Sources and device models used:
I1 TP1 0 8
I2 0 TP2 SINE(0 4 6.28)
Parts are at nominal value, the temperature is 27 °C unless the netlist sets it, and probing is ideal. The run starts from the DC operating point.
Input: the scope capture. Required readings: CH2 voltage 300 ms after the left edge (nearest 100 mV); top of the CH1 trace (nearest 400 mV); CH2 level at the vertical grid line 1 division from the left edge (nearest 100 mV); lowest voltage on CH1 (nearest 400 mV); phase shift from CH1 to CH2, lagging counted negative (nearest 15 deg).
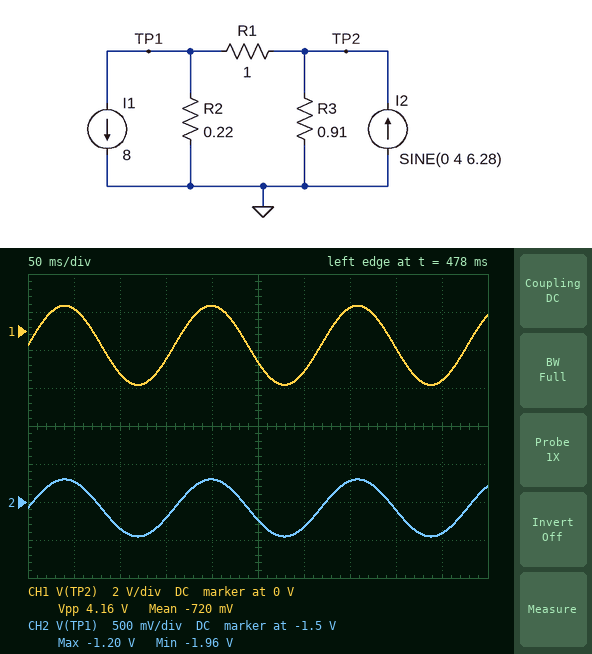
-1.8 V
1.2 V
-1.2 V
-2.8 V
0 deg
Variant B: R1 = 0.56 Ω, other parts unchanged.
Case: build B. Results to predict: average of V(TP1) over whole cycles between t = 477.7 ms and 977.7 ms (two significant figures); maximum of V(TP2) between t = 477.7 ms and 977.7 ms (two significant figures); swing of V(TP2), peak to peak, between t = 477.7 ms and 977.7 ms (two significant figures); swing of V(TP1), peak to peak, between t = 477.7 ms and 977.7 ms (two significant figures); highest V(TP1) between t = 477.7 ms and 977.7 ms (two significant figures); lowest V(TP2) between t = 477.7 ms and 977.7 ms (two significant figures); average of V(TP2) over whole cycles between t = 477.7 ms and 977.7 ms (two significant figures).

-1.5 V
730 mV
3.4 V
950 mV
-1.1 V
-2.6 V
-950 mV
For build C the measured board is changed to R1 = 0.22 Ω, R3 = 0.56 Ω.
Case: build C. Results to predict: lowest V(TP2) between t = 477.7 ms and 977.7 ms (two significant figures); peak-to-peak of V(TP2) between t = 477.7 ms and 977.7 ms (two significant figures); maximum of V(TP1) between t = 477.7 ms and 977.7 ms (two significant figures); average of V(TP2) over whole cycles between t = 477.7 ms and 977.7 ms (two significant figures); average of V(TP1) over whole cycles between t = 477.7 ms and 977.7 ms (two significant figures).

-2.0 V
2.0 V
-880 mV
-990 mV
-1.4 V
